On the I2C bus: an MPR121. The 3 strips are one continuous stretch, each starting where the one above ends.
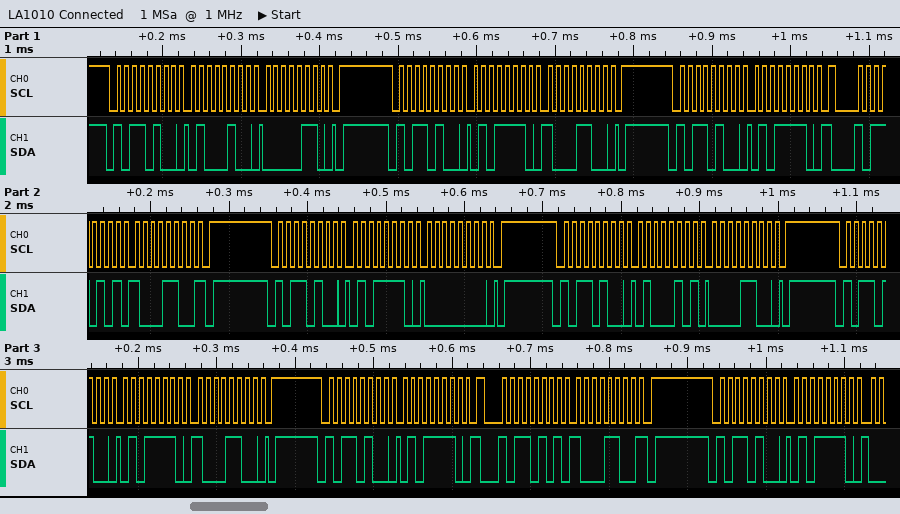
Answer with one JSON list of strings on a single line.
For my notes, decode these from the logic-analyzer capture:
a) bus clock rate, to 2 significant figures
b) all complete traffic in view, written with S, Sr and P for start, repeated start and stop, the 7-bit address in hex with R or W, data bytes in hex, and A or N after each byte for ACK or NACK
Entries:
["100 kHz", "S 5AW A 44 A 06 A P S 5AW A 5E A 8C A P S 5AW A 5E A Sr 5AR A 8C N P S 5AW A 5E A 00 A P S 5AW A 45 A 0C A P S 5AW A 5E A 8C A P S 5AW A 5E A Sr 5AR A 8C N P S 5AW A 5E A"]
